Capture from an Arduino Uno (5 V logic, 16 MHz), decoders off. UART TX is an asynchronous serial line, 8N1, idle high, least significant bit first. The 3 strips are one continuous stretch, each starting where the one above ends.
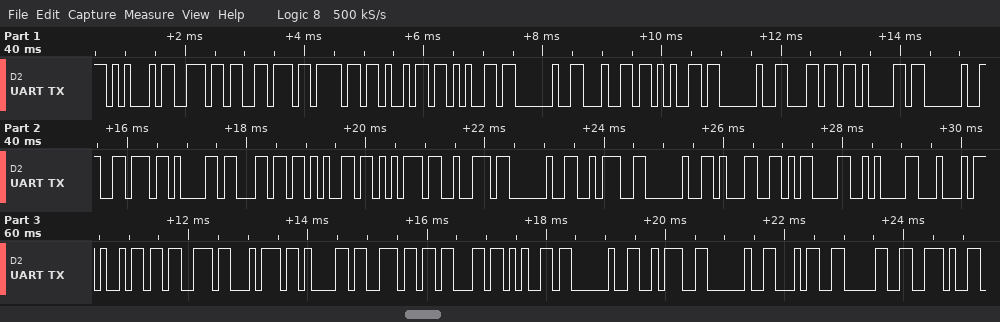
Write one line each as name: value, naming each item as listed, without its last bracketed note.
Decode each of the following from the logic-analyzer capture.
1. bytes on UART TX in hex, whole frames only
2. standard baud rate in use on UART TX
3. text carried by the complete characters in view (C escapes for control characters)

bytes on UART TX in hex, whole frames only: 45 6E 76 6F 69 65 20 64 65 20 6C 61 20 76 61 6C 65 75 72 20 3A 20 31 0D 0A 44 69 73 74 61 6E 63 65 20 3A 20 34 30 2E
standard baud rate in use on UART TX: 9600 baud
text carried by the complete characters in view: "Envoie de la valeur : 1\r\nDistance : 40."
